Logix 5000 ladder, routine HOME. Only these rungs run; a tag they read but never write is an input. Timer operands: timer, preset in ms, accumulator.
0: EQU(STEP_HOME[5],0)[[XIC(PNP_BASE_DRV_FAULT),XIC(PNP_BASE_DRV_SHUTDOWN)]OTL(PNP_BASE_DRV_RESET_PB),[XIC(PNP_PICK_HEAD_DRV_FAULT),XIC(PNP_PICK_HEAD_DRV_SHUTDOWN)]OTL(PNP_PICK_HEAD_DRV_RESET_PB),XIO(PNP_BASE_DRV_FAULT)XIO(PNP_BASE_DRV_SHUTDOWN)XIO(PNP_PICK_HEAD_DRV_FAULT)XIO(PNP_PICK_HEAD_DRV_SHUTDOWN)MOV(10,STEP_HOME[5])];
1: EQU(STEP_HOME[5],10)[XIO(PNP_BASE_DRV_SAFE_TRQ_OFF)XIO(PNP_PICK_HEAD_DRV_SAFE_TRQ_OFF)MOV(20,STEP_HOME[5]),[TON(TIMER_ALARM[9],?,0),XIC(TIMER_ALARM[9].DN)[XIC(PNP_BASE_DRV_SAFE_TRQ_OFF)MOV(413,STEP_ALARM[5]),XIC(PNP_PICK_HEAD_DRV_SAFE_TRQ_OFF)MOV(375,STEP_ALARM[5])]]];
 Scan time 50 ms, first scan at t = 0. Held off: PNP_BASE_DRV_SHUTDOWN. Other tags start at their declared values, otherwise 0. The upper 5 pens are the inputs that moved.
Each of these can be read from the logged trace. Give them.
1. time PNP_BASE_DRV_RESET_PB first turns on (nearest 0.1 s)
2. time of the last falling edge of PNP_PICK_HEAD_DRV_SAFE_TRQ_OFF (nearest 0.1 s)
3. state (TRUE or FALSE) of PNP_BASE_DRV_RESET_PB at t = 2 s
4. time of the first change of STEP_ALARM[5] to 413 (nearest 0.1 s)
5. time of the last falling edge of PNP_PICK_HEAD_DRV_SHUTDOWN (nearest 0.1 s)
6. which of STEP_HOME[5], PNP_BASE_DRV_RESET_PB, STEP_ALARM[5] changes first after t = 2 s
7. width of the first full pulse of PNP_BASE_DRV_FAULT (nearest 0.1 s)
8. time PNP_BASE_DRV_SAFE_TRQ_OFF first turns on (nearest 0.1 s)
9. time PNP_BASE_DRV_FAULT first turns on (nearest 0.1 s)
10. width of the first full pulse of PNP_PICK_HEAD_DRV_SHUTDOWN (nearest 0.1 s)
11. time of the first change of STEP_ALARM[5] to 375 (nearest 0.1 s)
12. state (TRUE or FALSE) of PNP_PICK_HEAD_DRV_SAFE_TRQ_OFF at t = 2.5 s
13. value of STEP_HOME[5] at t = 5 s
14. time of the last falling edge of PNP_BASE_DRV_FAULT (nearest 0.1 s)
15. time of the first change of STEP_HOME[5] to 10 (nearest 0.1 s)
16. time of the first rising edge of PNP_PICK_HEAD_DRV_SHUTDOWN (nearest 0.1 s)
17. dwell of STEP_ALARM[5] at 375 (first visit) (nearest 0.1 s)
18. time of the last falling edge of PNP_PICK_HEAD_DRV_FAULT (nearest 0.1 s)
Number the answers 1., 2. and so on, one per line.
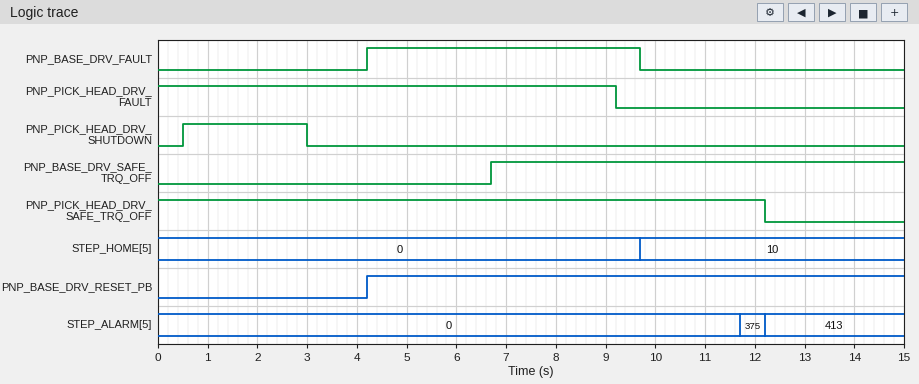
1. 4.2 s
2. 12.2 s
3. FALSE
4. 12.2 s
5. 3.0 s
6. PNP_BASE_DRV_RESET_PB
7. 5.5 s
8. 6.7 s
9. 4.2 s
10. 2.5 s
11. 11.7 s
12. TRUE
13. 0
14. 9.7 s
15. 9.7 s
16. 0.5 s
17. 0.5 s
18. 9.2 s
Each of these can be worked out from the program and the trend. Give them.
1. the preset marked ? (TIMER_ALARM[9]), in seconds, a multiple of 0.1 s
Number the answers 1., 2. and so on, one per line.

1. 2.0 s
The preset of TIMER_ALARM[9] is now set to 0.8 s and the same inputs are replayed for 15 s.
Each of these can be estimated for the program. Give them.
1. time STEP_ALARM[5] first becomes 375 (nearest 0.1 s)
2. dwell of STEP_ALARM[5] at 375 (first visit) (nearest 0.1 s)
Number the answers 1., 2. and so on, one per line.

1. 10.5 s
2. 1.7 s
